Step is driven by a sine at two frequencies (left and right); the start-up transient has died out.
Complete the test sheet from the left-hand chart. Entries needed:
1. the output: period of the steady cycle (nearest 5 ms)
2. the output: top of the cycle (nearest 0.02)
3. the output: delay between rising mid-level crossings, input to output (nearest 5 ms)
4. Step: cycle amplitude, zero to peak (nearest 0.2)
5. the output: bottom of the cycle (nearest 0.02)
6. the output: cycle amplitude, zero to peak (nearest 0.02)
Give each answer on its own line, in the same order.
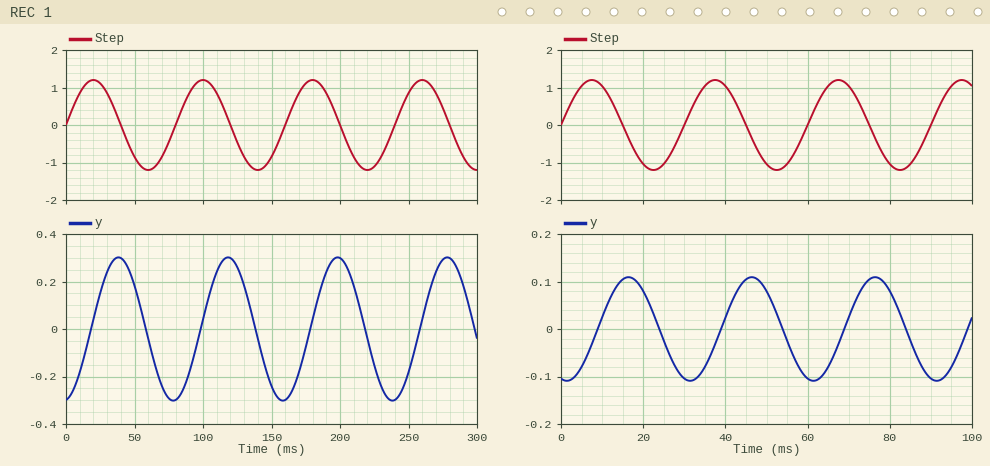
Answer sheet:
80 ms
0.30
20 ms
1.2
-0.30
0.30
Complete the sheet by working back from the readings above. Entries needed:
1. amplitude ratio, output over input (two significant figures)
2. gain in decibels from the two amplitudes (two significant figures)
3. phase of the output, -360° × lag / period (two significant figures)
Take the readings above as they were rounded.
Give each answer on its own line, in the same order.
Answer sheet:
0.25
-12 dB
-90°
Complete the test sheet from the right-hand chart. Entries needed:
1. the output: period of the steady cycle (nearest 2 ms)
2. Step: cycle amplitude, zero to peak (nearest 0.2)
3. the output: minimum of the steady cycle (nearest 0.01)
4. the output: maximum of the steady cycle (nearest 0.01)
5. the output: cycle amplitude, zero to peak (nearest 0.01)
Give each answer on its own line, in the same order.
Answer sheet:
30 ms
1.2
-0.11
0.11
0.11
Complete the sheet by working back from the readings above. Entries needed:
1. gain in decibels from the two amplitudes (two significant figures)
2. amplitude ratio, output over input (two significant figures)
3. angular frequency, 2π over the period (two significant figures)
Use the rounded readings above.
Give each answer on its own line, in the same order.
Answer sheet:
-21 dB
0.092
0.21 rad/ms
